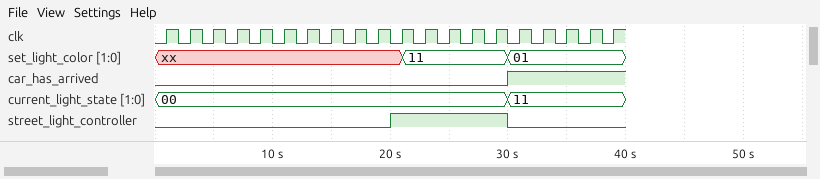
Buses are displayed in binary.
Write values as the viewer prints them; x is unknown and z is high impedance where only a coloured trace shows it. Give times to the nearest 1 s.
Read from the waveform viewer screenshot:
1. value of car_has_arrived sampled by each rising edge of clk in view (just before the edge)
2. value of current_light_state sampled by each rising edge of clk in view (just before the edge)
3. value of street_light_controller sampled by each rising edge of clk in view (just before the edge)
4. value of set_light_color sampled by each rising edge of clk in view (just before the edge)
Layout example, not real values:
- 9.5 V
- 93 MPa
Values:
- 0 0 0 0 0 0 0 0 0 0 0 0 0 0 0 1 1 1 1 1
- 00, 00, 00, 00, 00, 00, 00, 00, 00, 00, 00, 00, 00, 00, 00, 11, 11, 11, 11, 11
- 0 0 0 0 0 0 0 0 0 0 1 1 1 1 1 0 0 0 0 0
- xx, xx, xx, xx, xx, xx, xx, xx, xx, xx, xx, 11, 11, 11, 11, 01, 01, 01, 01, 01
